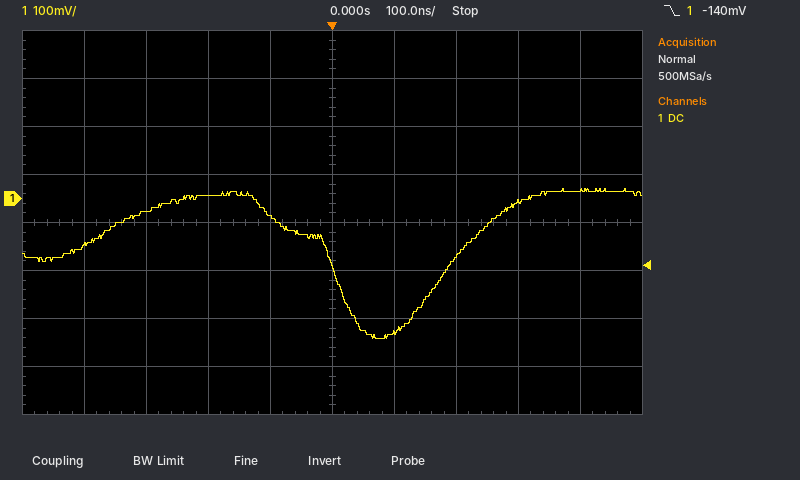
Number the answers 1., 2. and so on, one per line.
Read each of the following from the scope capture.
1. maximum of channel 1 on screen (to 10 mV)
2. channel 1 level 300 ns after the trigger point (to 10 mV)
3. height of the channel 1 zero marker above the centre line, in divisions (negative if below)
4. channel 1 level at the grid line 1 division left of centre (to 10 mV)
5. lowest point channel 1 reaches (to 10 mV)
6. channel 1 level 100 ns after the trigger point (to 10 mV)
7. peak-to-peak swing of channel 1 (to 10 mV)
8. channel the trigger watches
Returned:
1. 20 mV
2. -10 mV
3. +0.5 div
4. -40 mV
5. -290 mV
6. -280 mV
7. 310 mV
8. channel 1
